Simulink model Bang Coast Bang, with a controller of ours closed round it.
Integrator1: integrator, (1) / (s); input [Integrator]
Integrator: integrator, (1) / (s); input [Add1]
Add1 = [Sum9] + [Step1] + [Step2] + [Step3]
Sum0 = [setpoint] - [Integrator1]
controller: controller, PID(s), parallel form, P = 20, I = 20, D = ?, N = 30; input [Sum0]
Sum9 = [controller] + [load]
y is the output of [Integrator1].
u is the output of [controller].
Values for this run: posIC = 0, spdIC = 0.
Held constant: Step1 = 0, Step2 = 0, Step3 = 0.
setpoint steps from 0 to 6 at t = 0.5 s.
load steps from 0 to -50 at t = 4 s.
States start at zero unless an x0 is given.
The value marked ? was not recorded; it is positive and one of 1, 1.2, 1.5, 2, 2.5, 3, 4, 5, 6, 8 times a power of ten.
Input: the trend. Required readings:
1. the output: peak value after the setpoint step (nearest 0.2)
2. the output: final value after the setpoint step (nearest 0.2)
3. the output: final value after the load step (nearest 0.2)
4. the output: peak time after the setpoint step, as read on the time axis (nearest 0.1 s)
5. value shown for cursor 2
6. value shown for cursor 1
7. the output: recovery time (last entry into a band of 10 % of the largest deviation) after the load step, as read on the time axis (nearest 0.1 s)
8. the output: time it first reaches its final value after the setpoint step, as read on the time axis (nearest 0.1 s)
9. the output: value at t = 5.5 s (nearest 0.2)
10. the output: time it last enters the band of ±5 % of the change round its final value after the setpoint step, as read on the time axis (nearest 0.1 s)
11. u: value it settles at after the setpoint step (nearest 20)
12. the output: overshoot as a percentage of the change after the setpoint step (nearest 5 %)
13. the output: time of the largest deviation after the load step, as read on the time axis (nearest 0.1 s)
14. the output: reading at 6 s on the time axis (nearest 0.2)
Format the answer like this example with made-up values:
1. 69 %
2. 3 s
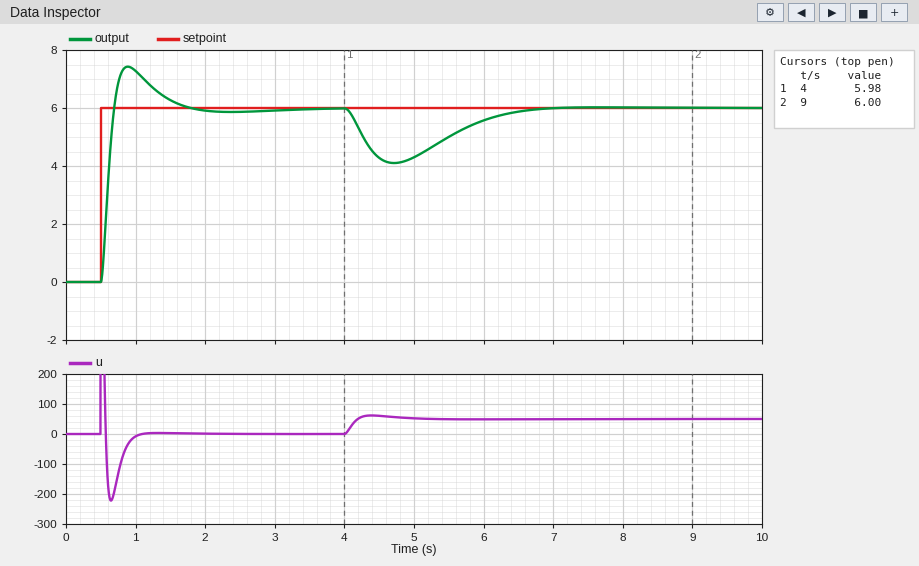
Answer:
1. 7.4
2. 6.0
3. 6.0
4. 0.9 s
5. 6.00
6. 5.98
7. 6.4 s
8. 0.7 s
9. 5.0
10. 1.5 s
11. 0
12. 25 %
13. 4.7 s
14. 5.6
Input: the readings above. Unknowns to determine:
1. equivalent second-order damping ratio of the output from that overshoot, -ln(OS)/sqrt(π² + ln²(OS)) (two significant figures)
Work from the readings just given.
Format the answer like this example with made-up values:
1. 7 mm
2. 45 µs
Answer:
1. 0.40
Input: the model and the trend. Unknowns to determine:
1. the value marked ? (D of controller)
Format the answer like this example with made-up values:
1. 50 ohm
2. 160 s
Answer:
1. 8
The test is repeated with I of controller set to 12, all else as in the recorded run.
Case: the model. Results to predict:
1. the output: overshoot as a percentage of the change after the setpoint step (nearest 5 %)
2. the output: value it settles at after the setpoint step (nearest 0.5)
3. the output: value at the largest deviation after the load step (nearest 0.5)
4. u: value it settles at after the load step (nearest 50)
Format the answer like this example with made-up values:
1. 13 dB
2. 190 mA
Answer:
1. 20 %
2. 6.0
3. 4.0
4. 50
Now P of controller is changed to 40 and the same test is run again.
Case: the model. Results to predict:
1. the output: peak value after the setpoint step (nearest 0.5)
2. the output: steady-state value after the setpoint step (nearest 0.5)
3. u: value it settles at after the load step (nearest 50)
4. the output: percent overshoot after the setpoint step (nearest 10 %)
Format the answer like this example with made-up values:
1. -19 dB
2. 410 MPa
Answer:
1. 8.0
2. 6.0
3. 50
4. 30 %
